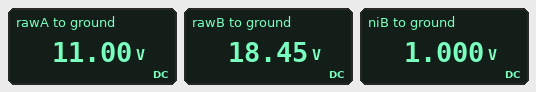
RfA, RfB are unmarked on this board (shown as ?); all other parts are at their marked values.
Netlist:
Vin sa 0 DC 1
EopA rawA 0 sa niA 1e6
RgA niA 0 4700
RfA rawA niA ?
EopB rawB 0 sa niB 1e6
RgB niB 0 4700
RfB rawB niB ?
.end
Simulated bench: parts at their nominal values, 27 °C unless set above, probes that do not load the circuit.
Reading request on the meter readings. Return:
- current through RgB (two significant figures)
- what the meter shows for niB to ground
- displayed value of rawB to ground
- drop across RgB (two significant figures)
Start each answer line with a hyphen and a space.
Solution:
- 210 µA
- 1.000 V
- 18.45 V
- 1.0 V
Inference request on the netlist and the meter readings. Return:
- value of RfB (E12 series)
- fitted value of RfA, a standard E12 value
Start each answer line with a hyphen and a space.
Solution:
- 82 kΩ
- 47 kΩ
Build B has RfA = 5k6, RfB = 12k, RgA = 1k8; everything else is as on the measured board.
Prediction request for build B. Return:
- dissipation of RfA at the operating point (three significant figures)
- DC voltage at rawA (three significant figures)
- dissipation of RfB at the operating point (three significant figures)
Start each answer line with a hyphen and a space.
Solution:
- 1.73 mW
- 4.11 V
- 543 µW
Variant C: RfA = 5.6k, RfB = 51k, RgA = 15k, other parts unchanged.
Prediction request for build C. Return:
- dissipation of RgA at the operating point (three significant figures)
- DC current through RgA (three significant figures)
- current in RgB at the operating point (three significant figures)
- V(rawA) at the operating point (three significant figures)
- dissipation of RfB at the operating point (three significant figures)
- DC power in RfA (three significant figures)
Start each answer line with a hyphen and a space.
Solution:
- 66.7 µW
- 66.7 µA
- 213 µA
- 1.37 V
- 2.31 mW
- 24.9 µW
